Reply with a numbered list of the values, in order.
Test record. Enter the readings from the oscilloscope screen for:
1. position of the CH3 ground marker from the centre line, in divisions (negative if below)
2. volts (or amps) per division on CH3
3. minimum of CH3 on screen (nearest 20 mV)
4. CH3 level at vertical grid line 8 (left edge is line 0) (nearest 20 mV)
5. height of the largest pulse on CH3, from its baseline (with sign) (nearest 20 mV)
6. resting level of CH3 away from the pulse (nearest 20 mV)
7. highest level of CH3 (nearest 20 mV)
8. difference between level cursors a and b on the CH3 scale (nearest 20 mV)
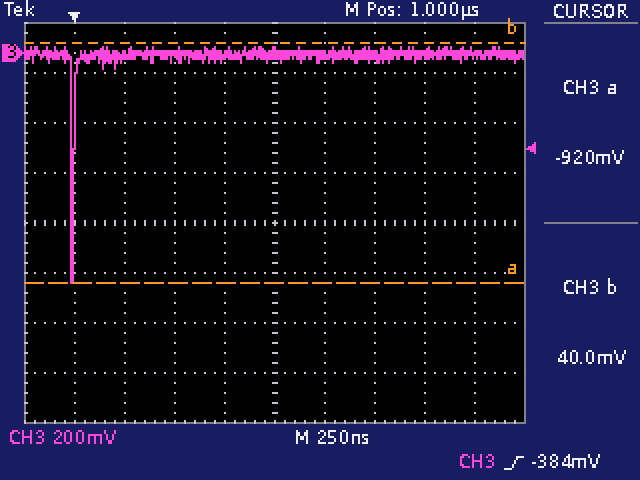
1. +3.4 div
2. 200 mV
3. -920 mV
4. 0 mV
5. -920 mV
6. 0 mV
7. 20 mV
8. 960 mV
